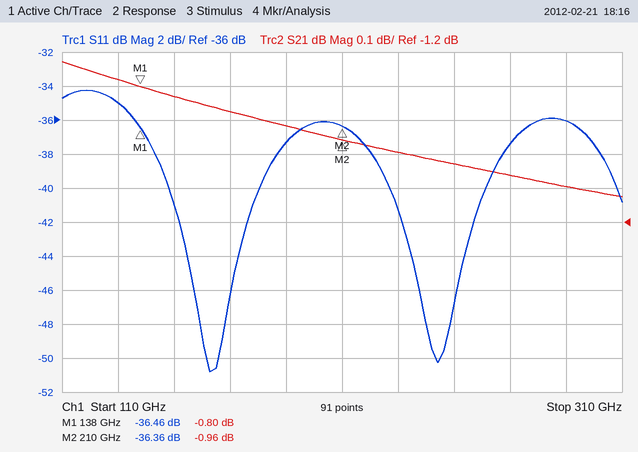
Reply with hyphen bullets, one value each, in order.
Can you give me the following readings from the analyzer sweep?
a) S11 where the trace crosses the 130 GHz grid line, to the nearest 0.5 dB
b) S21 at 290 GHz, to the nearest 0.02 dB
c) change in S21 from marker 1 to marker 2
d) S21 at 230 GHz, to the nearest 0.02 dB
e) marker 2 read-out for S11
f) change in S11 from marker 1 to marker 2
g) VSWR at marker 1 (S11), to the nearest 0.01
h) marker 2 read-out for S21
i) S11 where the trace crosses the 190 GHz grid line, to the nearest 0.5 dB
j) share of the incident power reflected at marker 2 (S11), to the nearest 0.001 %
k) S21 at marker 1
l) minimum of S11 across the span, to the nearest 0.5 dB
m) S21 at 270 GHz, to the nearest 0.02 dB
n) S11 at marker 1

- -35.0 dB
- -1.10 dB
- -0.16 dB
- -1.00 dB
- -36.36 dB
- 0.10 dB
- 1.03
- -0.96 dB
- -37.5 dB
- 0.023 %
- -0.80 dB
- -51.0 dB
- -1.06 dB
- -36.46 dB
